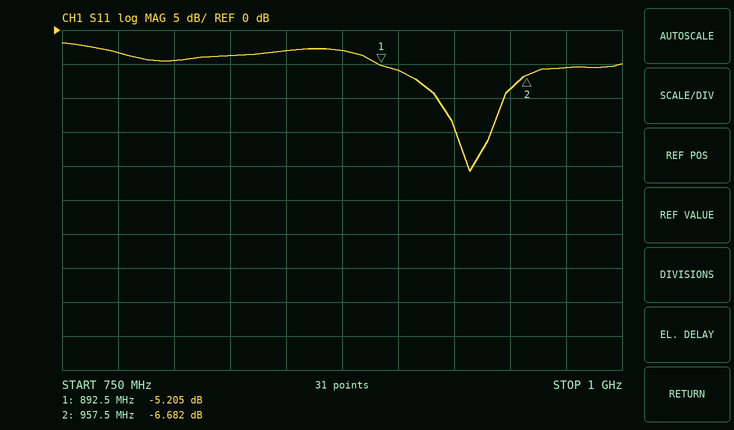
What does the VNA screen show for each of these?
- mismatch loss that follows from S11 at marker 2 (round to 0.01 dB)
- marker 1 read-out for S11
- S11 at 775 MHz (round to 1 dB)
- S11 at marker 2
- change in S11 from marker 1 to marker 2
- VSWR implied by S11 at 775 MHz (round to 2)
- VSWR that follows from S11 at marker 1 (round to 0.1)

1.05 dB
-5.205 dB
-3 dB
-6.682 dB
-1.477 dB
6
3.4
